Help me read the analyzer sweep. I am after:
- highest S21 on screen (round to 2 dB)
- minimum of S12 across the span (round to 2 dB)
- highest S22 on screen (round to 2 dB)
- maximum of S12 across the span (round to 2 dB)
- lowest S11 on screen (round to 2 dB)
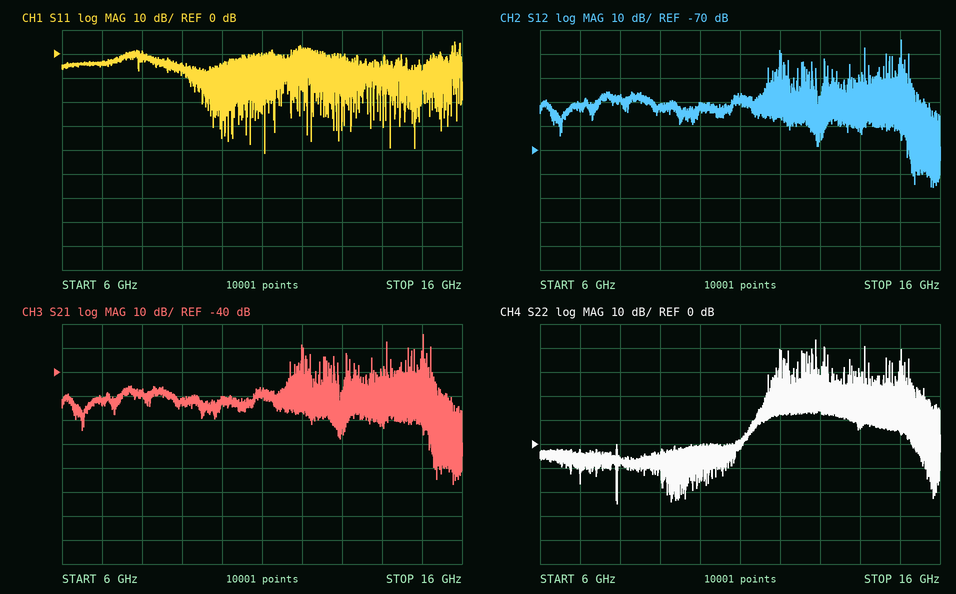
-24 dB
-86 dB
44 dB
-24 dB
-42 dB
